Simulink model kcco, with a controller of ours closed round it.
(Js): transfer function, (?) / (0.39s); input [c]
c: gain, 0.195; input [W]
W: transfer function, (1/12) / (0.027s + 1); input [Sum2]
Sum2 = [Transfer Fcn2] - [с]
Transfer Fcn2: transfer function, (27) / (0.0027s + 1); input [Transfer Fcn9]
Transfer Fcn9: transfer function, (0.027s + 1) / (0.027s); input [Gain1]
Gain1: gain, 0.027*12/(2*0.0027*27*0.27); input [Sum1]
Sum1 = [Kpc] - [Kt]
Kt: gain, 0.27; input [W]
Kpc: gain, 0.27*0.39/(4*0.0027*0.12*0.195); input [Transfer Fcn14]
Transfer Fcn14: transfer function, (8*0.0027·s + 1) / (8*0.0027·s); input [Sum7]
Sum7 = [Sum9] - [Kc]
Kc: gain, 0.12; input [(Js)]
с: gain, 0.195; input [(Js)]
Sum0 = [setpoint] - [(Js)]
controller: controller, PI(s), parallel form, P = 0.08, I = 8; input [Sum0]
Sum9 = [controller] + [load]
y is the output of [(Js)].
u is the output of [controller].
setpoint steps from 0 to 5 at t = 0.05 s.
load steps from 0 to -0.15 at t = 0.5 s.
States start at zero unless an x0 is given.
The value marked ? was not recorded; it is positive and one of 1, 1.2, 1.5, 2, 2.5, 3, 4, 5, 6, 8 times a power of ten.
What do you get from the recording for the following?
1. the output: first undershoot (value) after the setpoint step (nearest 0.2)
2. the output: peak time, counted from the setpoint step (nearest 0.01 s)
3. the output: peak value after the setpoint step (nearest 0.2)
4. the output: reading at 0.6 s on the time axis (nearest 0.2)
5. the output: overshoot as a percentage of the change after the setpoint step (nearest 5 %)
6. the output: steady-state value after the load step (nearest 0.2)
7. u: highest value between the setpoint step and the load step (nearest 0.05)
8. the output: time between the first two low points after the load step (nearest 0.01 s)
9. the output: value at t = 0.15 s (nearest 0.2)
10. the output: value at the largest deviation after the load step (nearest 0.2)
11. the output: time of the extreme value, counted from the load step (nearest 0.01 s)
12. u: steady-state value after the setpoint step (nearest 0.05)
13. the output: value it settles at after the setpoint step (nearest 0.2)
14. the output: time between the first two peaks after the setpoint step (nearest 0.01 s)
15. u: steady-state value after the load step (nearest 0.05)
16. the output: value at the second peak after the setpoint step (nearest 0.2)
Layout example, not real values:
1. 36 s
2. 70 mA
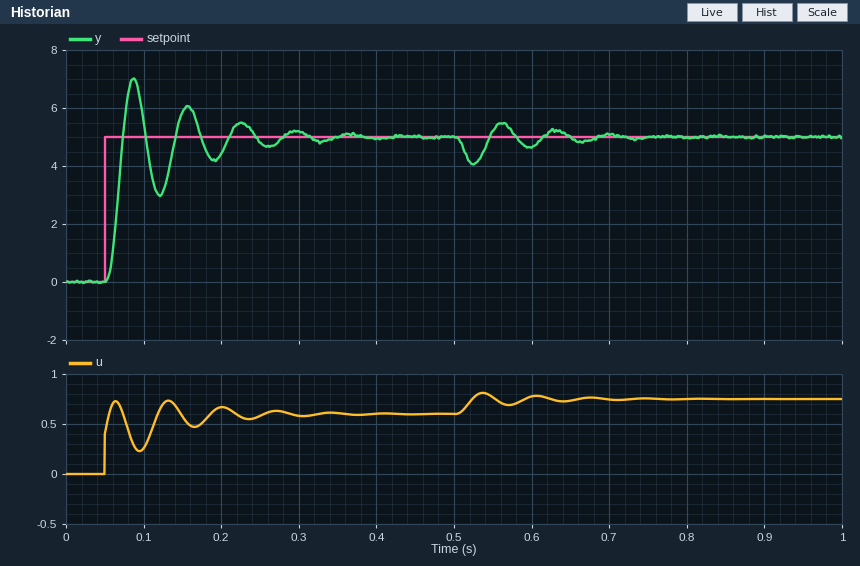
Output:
1. 3.0
2. 0.04 s
3. 7.0
4. 4.6
5. 40 %
6. 5.0
7. 0.75
8. 0.07 s
9. 5.8
10. 4.0
11. 0.03 s
12. 0.60
13. 5.0
14. 0.07 s
15. 0.75
16. 6.0
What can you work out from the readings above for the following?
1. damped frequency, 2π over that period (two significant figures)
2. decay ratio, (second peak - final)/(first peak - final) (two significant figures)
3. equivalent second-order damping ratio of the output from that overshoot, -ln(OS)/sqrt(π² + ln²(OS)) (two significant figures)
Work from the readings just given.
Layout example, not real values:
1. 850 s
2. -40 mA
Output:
1. 90 rad/s
2. 0.50
3. 0.28
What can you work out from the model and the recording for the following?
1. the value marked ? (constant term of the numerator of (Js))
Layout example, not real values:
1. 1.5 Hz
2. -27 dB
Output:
1. 0.5
